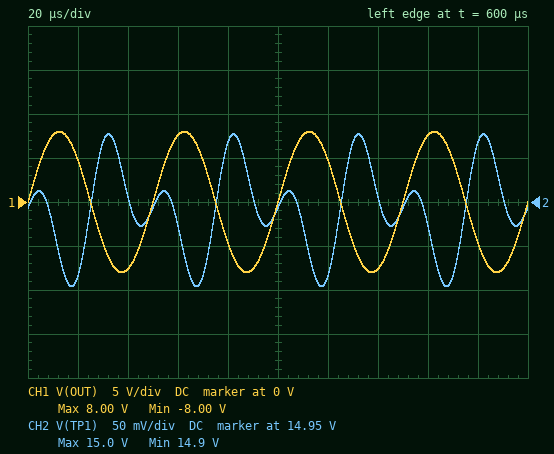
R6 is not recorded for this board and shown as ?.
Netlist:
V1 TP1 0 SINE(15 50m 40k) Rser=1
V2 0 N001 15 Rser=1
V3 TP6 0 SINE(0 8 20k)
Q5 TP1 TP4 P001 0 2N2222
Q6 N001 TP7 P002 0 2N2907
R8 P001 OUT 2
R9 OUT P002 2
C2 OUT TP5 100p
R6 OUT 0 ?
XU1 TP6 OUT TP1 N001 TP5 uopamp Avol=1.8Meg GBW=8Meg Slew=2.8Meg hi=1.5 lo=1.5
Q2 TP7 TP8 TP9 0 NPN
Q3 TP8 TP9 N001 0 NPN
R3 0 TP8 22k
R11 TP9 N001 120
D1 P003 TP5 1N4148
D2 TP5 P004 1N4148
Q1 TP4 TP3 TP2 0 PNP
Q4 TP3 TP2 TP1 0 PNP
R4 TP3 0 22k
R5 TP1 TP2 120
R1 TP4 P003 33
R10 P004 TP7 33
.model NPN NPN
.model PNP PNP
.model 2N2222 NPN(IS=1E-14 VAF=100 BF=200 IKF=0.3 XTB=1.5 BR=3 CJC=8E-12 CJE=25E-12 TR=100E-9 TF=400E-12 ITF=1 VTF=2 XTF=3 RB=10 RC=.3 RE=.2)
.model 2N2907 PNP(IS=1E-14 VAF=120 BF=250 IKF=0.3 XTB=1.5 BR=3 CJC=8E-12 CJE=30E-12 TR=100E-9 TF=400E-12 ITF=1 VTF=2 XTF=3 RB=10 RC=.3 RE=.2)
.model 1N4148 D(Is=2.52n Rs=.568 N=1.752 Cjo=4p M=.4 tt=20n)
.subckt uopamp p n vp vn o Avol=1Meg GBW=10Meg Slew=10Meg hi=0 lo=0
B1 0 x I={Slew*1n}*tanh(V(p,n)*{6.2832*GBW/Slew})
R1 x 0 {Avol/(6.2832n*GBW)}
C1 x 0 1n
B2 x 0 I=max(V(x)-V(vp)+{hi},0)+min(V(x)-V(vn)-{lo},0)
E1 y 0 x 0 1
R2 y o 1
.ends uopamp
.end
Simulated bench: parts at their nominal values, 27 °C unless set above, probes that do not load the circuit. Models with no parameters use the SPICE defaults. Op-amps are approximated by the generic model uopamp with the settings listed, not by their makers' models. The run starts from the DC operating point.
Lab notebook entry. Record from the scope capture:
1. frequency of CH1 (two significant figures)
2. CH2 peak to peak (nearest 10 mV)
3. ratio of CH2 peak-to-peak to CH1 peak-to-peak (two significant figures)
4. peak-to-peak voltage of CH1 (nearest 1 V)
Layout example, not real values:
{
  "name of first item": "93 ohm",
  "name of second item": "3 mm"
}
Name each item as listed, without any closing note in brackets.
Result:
{
  "frequency of CH1": "20 kHz",
  "CH2 peak to peak": "170 mV",
  "ratio of CH2 peak-to-peak to CH1 peak-to-peak": "0.011",
  "peak-to-peak voltage of CH1": "16 V"
}
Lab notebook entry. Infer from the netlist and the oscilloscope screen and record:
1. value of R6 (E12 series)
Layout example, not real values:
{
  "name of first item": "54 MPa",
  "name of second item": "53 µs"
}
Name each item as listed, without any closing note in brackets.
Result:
{
  "value of R6": "82 Ω"
}
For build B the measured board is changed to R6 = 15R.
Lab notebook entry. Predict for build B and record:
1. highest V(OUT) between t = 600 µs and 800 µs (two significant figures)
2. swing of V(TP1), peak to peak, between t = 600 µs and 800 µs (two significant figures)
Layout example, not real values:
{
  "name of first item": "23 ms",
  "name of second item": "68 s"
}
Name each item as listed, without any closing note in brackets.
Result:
{
  "highest V(OUT) between t = 600 µs and 800 µs": "7.7 V",
  "swing of V(TP1), peak to peak, between t = 600 µs and 800 µs": "590 mV"
}
